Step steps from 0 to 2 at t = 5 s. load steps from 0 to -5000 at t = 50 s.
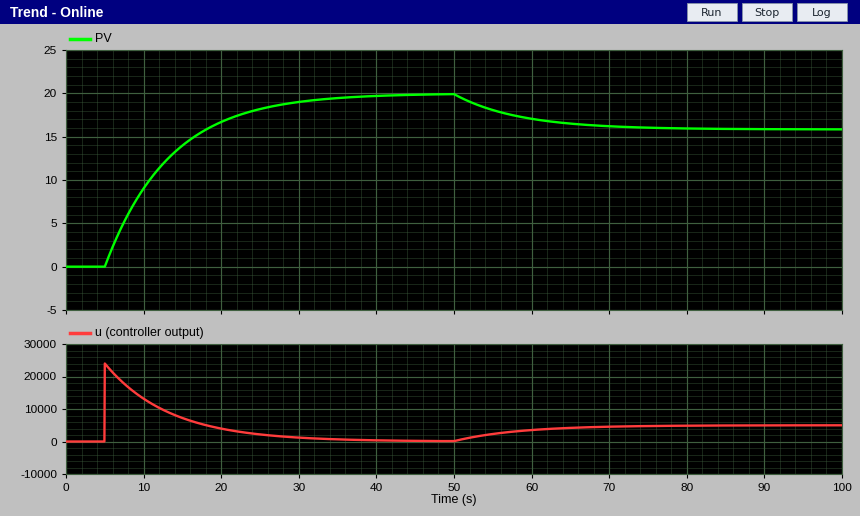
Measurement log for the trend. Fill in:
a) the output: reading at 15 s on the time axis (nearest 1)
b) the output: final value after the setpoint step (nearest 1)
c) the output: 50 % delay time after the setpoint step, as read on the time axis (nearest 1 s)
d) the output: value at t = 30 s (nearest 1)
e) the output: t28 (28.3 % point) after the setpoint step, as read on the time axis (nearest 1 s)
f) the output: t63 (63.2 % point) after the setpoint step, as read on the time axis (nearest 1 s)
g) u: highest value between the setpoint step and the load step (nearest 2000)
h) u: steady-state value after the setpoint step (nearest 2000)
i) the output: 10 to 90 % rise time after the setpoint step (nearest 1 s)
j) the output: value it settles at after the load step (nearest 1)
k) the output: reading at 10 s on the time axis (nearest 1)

14
20
11 s
19
8 s
13 s
24000
0
18 s
16
9
